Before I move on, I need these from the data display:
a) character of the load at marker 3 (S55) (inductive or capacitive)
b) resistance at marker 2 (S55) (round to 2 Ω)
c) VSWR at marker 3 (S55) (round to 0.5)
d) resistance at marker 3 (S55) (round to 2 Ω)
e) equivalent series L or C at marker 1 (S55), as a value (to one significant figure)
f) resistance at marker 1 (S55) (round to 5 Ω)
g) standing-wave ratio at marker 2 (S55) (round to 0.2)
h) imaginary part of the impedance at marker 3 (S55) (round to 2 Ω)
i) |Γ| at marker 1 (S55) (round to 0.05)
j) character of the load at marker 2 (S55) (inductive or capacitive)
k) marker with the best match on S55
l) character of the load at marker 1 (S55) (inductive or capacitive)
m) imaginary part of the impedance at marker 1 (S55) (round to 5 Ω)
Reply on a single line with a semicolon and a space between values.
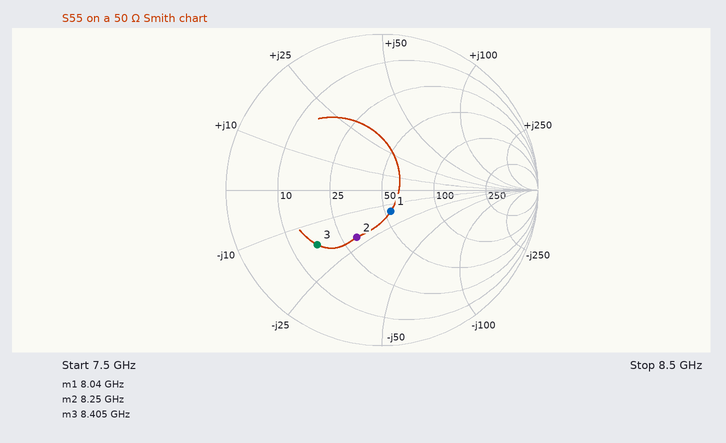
capacitive; 30 Ω; 3.5; 16 Ω; 1 pF; 55 Ω; 2.0; -16 Ω; 0.15; capacitive; marker 1; capacitive; -15 Ω
